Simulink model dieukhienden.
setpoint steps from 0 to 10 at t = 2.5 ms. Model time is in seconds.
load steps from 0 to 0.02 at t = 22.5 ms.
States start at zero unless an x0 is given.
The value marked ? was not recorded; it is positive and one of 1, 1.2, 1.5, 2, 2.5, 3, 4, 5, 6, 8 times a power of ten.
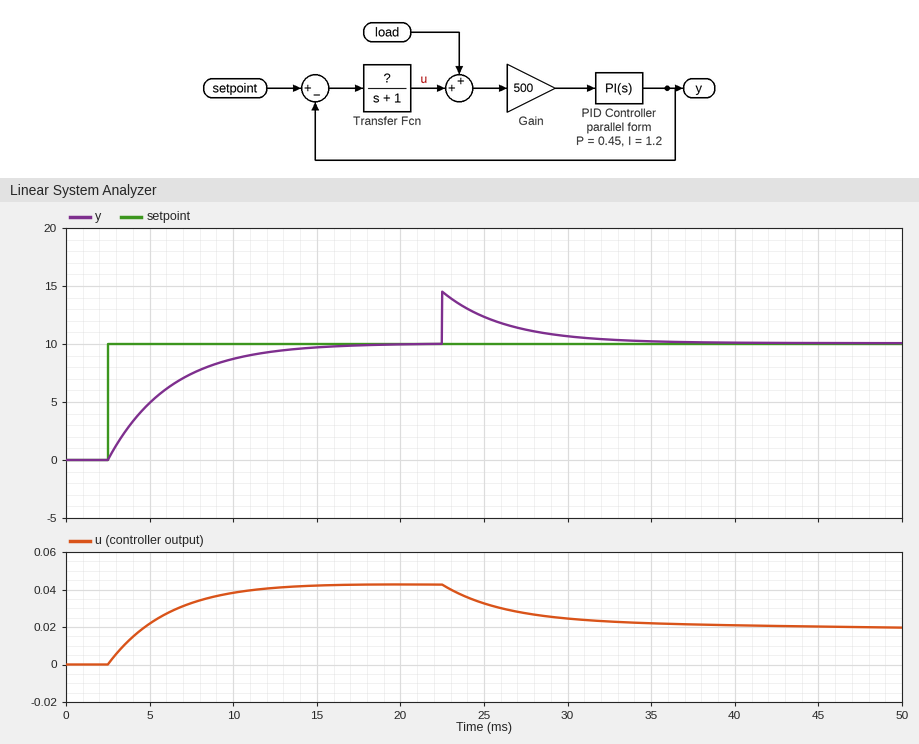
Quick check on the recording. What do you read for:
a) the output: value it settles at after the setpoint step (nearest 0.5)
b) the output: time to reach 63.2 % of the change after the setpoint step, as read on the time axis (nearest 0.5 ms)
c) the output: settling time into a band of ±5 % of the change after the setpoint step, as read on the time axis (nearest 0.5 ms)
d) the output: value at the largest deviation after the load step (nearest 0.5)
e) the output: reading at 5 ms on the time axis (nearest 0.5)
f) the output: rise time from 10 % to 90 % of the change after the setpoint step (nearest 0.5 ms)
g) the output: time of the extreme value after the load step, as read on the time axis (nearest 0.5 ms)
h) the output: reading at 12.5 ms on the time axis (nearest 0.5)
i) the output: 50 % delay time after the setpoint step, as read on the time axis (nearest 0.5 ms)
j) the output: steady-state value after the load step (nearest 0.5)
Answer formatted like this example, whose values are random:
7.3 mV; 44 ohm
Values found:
10.0; 6.0 ms; 13.5 ms; 14.5; 5.0; 8.0 ms; 22.5 ms; 9.5; 5.0 ms; 10.0
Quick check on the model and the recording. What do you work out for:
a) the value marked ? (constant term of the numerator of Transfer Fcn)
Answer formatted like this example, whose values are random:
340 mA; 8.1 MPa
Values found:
1.2
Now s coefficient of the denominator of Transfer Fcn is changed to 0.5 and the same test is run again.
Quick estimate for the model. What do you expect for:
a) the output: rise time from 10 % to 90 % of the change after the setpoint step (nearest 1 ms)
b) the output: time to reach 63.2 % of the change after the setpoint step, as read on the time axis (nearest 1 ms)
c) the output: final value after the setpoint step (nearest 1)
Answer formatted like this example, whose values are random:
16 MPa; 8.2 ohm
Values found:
4 ms; 4 ms; 10
